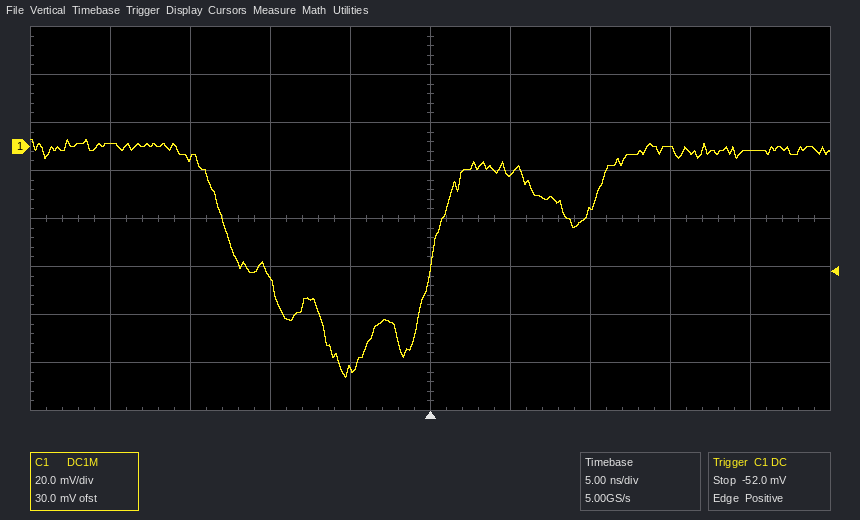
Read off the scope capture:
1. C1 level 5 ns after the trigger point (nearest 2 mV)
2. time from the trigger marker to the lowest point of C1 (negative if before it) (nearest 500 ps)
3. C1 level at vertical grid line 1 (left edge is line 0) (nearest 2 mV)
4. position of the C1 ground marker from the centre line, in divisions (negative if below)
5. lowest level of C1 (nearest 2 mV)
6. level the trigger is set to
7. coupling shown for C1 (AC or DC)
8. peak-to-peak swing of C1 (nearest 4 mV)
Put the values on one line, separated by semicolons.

-12 mV; -5.5 ns; 2 mV; +1.5 div; -96 mV; -52.0 mV; DC; 100 mV
